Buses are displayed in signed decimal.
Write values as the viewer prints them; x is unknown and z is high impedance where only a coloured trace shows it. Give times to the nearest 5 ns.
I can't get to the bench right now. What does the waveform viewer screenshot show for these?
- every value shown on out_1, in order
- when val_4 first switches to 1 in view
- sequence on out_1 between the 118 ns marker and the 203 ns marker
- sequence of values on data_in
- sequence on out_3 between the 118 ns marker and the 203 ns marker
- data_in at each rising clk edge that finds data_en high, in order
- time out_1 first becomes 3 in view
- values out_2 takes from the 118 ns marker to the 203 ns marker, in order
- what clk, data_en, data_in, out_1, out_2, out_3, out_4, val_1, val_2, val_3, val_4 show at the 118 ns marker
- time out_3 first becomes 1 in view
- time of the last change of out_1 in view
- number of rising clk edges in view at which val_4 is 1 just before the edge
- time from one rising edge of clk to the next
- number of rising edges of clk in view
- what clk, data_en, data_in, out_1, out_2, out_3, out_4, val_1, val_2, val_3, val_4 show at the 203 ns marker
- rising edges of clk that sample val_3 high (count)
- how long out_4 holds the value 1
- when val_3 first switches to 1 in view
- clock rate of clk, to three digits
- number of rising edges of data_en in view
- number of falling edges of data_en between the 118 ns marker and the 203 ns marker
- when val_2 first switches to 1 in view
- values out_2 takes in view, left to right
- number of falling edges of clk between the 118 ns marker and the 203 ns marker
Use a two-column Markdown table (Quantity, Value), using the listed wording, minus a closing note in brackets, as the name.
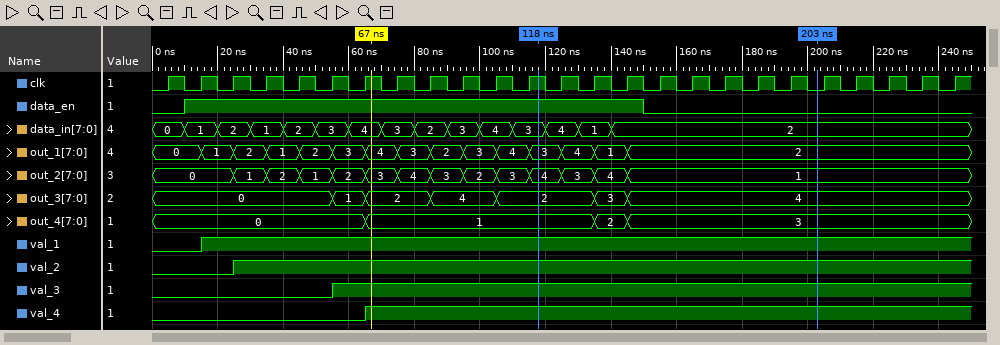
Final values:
| Quantity | Value |
|---|---|
| every value shown on out_1, in order | 0, 1, 2, 1, 2, 3, 4, 3, 2, 3, 4, 3, 4, 1, 2 |
| when val_4 first switches to 1 in view | 65 ns |
| sequence on out_1 between the 118 ns marker and the 203 ns marker | 3, 4, 1, 2 |
| sequence of values on data_in | 0, 1, 2, 1, 2, 3, 4, 3, 2, 3, 4, 3, 4, 1, 2 |
| sequence on out_3 between the 118 ns marker and the 203 ns marker | 2, 3, 4 |
| data_in at each rising clk edge that finds data_en high, in order | 1, 2, 1, 2, 3, 4, 3, 2, 3, 4, 3, 4, 1, 2 |
| time out_1 first becomes 3 in view | 55 ns |
| values out_2 takes from the 118 ns marker to the 203 ns marker, in order | 4, 3, 4, 1 |
| what clk, data_en, data_in, out_1, out_2, out_3, out_4, val_1, val_2, val_3, val_4 show at the 118 ns marker | clk=1, data_en=1, data_in=3, out_1=3, out_2=4, out_3=2, out_4=1, val_1=1, val_2=1, val_3=1, val_4=1 |
| time out_3 first becomes 1 in view | 55 ns |
| time of the last change of out_1 in view | 145 ns |
| number of rising clk edges in view at which val_4 is 1 just before the edge | 18 |
| time from one rising edge of clk to the next | 10 ns |
| number of rising edges of clk in view | 25 |
| what clk, data_en, data_in, out_1, out_2, out_3, out_4, val_1, val_2, val_3, val_4 show at the 203 ns marker | clk=0, data_en=0, data_in=2, out_1=2, out_2=1, out_3=4, out_4=3, val_1=1, val_2=1, val_3=1, val_4=1 |
| rising edges of clk that sample val_3 high | 19 |
| how long out_4 holds the value 1 | 70 ns |
| when val_3 first switches to 1 in view | 55 ns |
| clock rate of clk, to three digits | 100 MHz |
| number of rising edges of data_en in view | 1 |
| number of falling edges of data_en between the 118 ns marker and the 203 ns marker | 1 |
| when val_2 first switches to 1 in view | 25 ns |
| values out_2 takes in view, left to right | 0, 1, 2, 1, 2, 3, 4, 3, 2, 3, 4, 3, 4, 1 |
| number of falling edges of clk between the 118 ns marker and the 203 ns marker | 9 |
